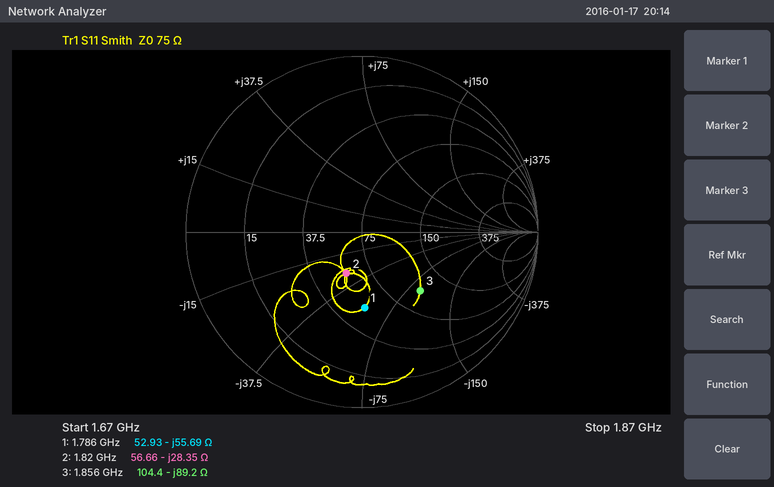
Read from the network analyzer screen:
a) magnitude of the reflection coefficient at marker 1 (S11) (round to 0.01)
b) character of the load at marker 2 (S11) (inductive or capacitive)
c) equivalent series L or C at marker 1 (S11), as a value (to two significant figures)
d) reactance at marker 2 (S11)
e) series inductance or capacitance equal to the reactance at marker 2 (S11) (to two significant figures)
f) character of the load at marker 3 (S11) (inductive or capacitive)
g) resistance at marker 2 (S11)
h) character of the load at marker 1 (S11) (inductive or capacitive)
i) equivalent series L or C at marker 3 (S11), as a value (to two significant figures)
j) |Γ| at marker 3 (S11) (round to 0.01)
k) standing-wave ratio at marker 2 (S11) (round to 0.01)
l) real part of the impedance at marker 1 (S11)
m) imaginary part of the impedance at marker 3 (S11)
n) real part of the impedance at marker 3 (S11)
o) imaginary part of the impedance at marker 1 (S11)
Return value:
0.43
capacitive
1.6 pF
-28.35 Ω
3.1 pF
capacitive
56.66 Ω
capacitive
960 fF
0.47
1.67
52.93 Ω
-89.2 Ω
104.4 Ω
-55.69 Ω
